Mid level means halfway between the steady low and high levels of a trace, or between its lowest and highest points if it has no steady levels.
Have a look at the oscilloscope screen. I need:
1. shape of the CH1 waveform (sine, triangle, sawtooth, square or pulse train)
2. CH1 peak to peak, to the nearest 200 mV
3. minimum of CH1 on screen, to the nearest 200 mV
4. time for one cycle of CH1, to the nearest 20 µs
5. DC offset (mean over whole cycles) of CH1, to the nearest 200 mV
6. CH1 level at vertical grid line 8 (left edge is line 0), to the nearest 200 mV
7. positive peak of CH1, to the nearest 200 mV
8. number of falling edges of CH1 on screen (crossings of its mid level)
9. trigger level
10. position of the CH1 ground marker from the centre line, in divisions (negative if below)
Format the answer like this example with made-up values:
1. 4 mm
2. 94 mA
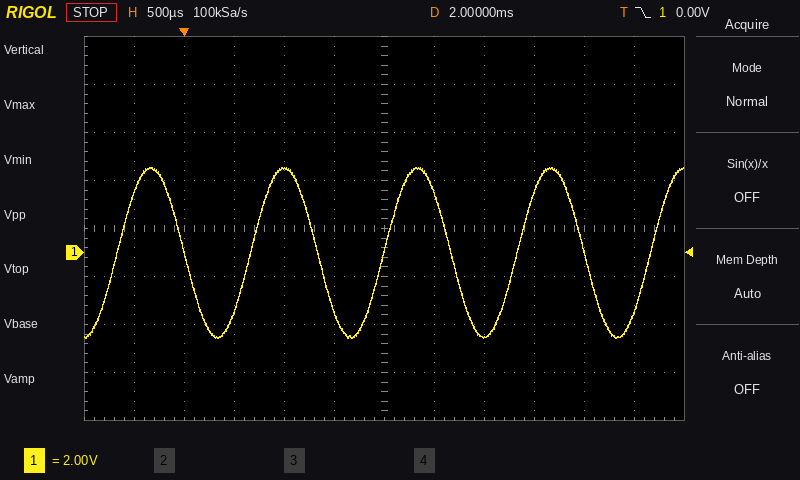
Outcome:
1. sine
2. 7.2 V
3. -3.6 V
4. 1.34 ms
5. 0.0 V
6. -3.6 V
7. 3.6 V
8. 4
9. 0.00 V
10. -0.5 div
